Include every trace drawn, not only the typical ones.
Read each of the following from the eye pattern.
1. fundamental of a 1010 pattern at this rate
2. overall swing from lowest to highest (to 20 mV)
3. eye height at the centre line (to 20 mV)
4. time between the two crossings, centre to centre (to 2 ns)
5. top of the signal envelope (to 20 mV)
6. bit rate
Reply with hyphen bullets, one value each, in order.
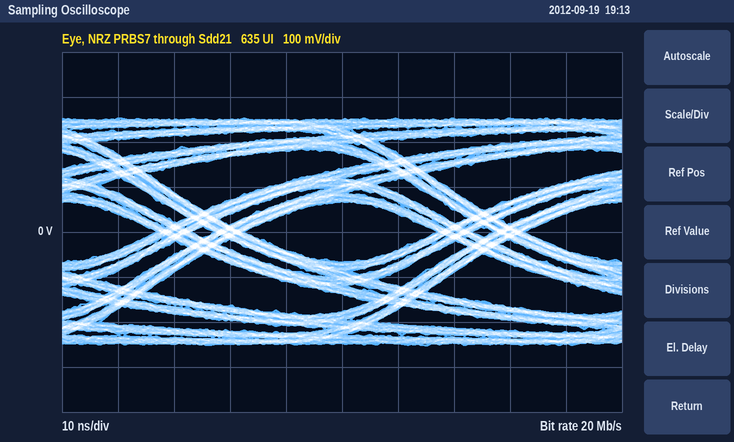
- 10 MHz
- 500 mV
- 140 mV
- 50 ns
- 260 mV
- 20 Mb/s
